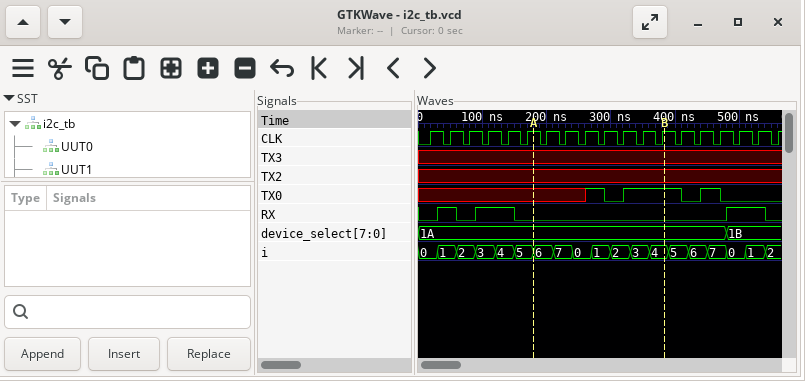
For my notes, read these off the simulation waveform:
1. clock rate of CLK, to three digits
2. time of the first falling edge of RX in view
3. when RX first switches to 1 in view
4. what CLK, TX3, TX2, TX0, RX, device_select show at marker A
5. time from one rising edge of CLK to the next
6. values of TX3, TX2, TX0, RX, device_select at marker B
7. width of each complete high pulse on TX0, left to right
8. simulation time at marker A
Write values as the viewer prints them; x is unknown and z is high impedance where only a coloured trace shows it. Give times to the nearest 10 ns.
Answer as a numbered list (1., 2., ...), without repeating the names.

1. 33.3 MHz
2. 60 ns
3. 30 ns
4. CLK=1, TX3=x, TX2=x, TX0=x, RX=0, device_select=1A
5. 30 ns
6. TX3=x, TX2=x, TX0=1, RX=0, device_select=1A
7. 90 ns, 30 ns
8. 180 ns
